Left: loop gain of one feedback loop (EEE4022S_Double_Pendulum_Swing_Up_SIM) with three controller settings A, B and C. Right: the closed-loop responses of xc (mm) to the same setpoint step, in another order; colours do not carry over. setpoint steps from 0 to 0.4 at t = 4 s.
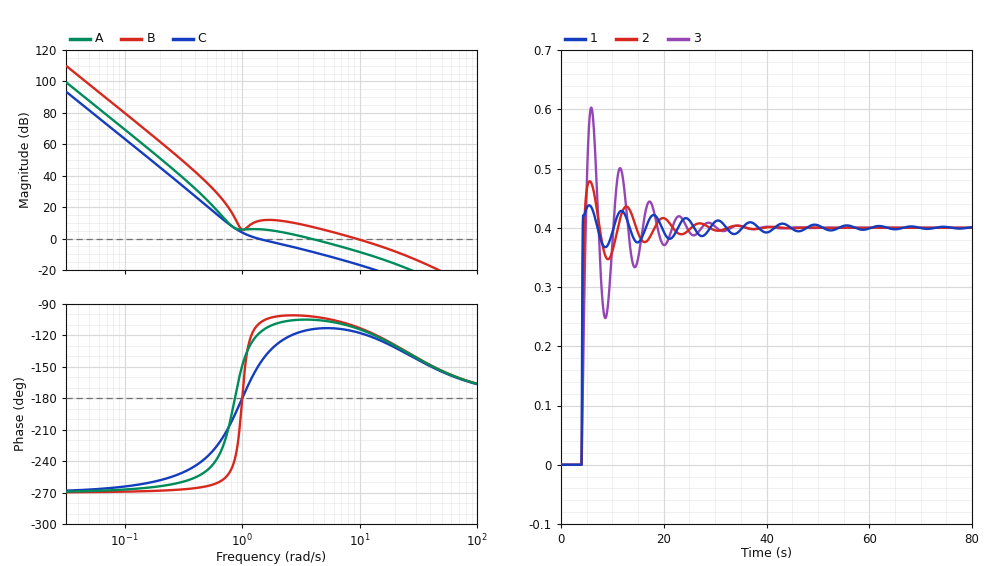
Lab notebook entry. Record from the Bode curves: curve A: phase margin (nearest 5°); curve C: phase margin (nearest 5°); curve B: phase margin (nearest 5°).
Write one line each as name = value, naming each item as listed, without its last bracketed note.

curve A: phase margin = 75°
curve C: phase margin = 30°
curve B: phase margin = 70°
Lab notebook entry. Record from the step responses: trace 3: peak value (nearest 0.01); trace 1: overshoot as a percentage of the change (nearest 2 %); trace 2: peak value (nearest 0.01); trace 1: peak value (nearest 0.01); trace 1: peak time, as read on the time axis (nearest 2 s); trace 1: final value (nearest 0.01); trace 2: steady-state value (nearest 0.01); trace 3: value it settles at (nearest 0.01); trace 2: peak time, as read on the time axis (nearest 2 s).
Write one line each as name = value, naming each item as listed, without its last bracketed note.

trace 3: peak value = 0.60
trace 1: overshoot as a percentage of the change = 10 %
trace 2: peak value = 0.48
trace 1: peak value = 0.44
trace 1: peak time, as read on the time axis = 6 s
trace 1: final value = 0.40
trace 2: steady-state value = 0.40
trace 3: value it settles at = 0.40
trace 2: peak time, as read on the time axis = 6 s
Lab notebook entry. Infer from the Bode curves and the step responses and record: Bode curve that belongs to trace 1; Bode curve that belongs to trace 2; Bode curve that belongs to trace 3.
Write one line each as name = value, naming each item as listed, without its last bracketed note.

Bode curve that belongs to trace 1 = B
Bode curve that belongs to trace 2 = A
Bode curve that belongs to trace 3 = C
